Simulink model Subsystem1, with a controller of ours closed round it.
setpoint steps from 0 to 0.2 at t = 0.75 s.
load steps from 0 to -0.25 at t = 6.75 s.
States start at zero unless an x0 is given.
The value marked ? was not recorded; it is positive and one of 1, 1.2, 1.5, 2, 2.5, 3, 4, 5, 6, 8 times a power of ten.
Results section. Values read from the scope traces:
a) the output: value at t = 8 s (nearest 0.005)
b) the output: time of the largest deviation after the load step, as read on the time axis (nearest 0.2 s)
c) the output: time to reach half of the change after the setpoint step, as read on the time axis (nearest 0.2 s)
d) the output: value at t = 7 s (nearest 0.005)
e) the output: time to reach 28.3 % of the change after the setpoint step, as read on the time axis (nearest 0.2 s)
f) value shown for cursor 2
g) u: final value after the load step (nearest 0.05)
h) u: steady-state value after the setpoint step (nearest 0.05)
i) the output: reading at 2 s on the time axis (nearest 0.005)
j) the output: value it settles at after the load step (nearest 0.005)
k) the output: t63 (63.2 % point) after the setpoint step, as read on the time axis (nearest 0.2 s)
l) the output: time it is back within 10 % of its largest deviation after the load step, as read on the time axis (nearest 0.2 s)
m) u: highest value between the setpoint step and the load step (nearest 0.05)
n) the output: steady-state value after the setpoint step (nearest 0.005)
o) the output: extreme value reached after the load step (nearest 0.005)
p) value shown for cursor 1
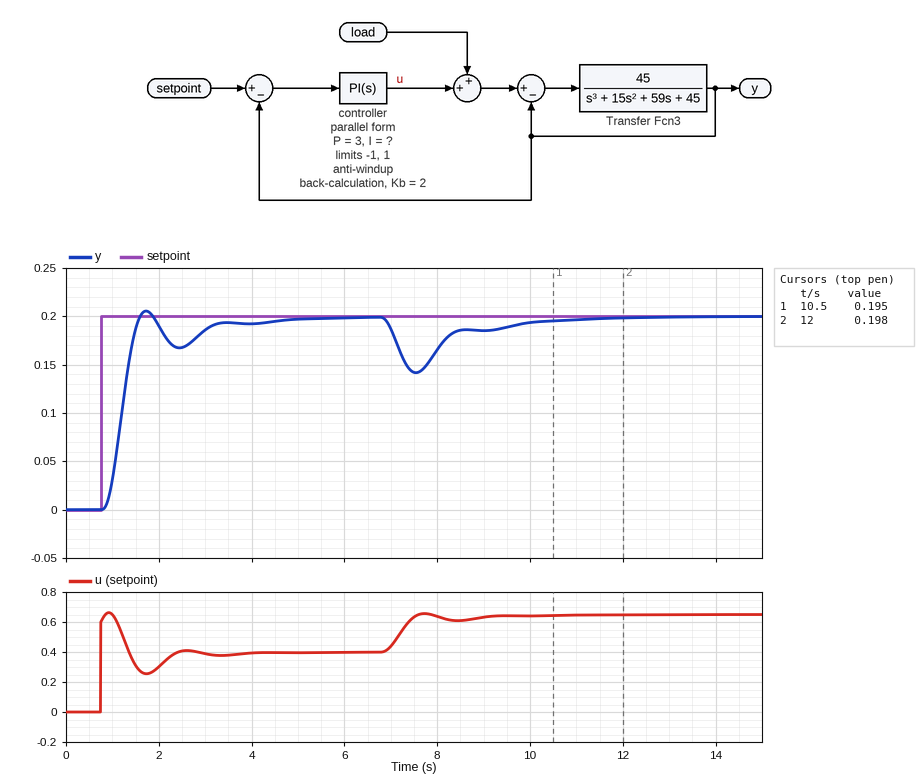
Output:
0.165
7.6 s
1.2 s
0.185
1.0 s
0.198
0.65
0.40
0.190
0.200
1.2 s
10.2 s
0.65
0.200
0.140
0.195
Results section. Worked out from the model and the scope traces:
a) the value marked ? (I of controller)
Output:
3
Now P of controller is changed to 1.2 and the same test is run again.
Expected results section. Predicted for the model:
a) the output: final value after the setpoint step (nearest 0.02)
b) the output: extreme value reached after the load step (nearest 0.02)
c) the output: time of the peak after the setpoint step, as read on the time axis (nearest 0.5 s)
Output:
0.20
0.12
2.5 s
